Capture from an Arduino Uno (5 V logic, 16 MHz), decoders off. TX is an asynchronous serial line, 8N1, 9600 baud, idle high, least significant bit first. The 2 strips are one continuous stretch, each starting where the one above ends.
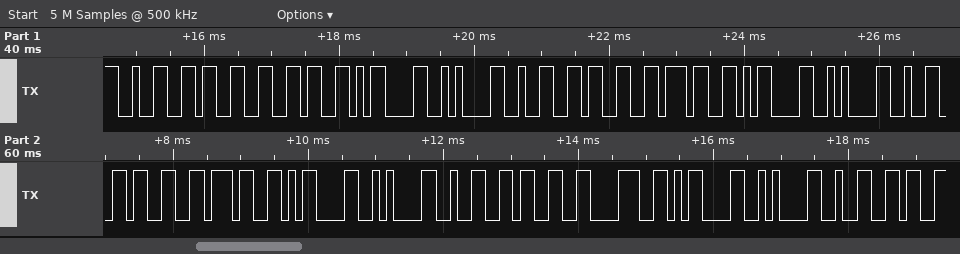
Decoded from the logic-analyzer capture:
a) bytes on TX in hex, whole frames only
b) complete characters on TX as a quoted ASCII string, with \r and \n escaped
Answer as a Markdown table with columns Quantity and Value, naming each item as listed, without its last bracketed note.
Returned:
| Quantity | Value |
|---|---|
| bytes on TX in hex, whole frames only | 0x32 0x33 0x36 0x0D 0x0A 0x32 0x33 0x37 0x0D 0x0A 0x32 0x33 0x37 0x0D 0x0A 0x32 0x33 0x38 0x0D 0x0A 0x32 |
| complete characters on TX as a quoted ASCII string, with \r and \n escaped | "236\r\n237\r\n237\r\n238\r\n2" |
